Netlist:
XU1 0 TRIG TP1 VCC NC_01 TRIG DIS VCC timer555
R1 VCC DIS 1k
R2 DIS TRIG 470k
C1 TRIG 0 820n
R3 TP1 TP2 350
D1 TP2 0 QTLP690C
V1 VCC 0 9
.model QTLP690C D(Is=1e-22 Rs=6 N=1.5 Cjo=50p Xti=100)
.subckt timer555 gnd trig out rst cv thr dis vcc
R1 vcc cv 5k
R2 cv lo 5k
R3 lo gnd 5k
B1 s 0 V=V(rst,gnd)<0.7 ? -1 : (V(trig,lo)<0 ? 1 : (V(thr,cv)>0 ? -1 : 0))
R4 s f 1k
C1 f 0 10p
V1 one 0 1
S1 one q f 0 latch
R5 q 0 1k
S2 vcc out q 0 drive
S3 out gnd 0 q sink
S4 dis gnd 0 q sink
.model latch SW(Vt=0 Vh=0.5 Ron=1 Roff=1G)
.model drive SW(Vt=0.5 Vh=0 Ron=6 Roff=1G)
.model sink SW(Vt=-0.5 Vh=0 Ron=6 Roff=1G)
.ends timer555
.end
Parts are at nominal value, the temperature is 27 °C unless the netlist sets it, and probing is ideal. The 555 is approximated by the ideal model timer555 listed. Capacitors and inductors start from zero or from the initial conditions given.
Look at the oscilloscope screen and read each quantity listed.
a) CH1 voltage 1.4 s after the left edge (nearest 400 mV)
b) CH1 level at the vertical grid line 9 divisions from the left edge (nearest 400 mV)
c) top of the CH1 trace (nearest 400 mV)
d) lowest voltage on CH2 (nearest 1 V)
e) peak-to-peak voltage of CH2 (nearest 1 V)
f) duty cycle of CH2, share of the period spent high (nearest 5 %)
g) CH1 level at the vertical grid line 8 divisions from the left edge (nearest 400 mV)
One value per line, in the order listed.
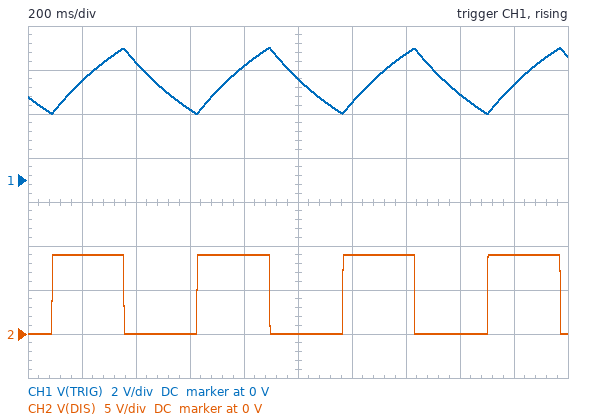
5.6 V
4.4 V
6.0 V
0 V
9 V
50 %
4.0 V
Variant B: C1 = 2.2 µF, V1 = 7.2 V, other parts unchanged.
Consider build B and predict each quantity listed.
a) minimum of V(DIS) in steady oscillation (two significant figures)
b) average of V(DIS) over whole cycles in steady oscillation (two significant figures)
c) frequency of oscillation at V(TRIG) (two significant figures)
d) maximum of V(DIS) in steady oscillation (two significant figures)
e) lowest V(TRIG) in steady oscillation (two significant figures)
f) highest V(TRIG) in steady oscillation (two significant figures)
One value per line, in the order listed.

43 mV
3.6 V
690 mHz
7.2 V
2.4 V
4.8 V
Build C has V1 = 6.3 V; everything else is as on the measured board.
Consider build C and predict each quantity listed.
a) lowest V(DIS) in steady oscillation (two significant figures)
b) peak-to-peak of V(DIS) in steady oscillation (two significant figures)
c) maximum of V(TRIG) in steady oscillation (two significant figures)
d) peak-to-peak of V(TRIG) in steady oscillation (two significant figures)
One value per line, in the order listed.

38 mV
6.3 V
4.2 V
2.1 V
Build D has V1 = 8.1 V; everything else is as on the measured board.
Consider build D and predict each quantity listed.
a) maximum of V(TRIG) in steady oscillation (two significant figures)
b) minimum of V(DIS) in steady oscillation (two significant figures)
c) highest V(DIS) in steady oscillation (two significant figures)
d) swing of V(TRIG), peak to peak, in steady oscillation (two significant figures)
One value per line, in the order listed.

5.4 V
48 mV
8.1 V
2.7 V
